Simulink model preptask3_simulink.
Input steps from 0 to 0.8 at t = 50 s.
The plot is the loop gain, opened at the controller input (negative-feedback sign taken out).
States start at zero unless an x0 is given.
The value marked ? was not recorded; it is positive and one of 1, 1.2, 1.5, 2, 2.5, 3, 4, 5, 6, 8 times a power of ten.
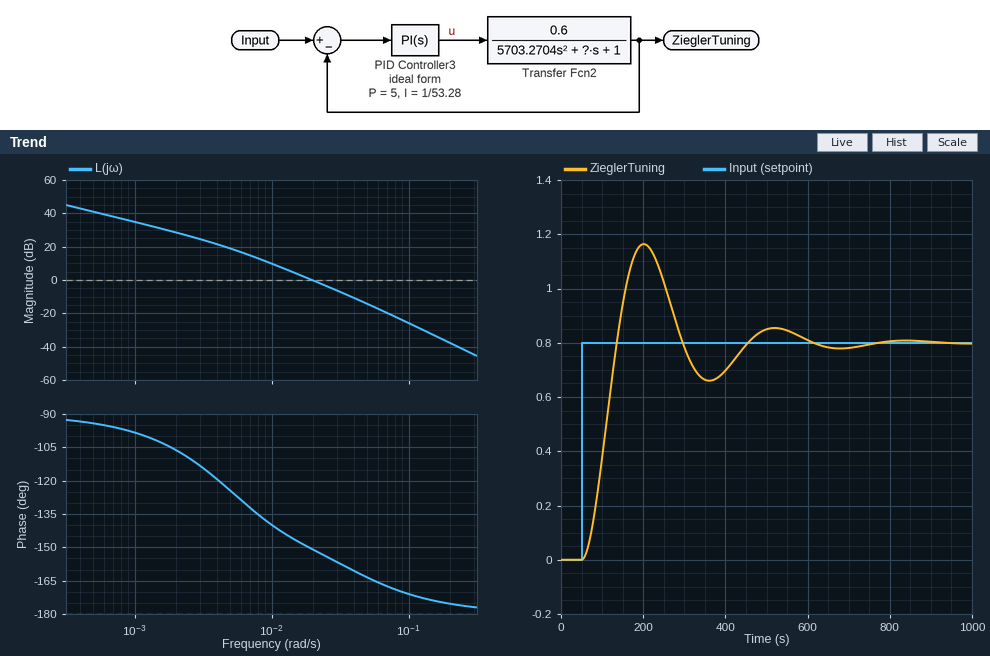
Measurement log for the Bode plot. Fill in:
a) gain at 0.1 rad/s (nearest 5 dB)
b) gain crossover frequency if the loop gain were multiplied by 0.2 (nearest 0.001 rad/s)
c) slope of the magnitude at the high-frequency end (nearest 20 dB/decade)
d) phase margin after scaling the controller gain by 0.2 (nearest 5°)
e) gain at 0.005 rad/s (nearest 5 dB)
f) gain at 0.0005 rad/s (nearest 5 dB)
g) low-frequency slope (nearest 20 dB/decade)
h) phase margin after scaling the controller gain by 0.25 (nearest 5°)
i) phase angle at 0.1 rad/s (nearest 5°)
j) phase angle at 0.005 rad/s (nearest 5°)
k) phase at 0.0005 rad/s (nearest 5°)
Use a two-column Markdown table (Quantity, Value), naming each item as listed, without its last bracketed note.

| Quantity | Value |
|---|---|
| gain at 0.1 rad/s | -25 dB |
| gain crossover frequency if the loop gain were multiplied by 0.2 | 0.007 rad/s |
| slope of the magnitude at the high-frequency end | -40 dB/decade |
| phase margin after scaling the controller gain by 0.2 | 45° |
| gain at 0.005 rad/s | 20 dB |
| gain at 0.0005 rad/s | 40 dB |
| low-frequency slope | -20 dB/decade |
| phase margin after scaling the controller gain by 0.25 | 45° |
| phase angle at 0.1 rad/s | -170° |
| phase angle at 0.005 rad/s | -125° |
| phase at 0.0005 rad/s | -95° |
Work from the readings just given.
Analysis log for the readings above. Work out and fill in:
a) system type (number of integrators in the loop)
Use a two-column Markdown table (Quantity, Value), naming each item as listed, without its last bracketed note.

| Quantity | Value |
|---|---|
| system type | 1 |
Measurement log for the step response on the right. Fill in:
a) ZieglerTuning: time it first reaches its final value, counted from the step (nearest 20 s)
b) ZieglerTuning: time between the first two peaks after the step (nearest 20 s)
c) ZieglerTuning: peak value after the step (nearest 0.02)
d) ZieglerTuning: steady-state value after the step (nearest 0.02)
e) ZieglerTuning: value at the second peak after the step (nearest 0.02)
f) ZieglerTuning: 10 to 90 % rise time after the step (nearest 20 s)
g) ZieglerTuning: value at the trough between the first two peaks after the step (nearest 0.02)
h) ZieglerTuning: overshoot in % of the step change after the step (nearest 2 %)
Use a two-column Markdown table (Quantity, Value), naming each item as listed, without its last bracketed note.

| Quantity | Value |
|---|---|
| ZieglerTuning: time it first reaches its final value, counted from the step | 80 s |
| ZieglerTuning: time between the first two peaks after the step | 320 s |
| ZieglerTuning: peak value after the step | 1.16 |
| ZieglerTuning: steady-state value after the step | 0.80 |
| ZieglerTuning: value at the second peak after the step | 0.86 |
| ZieglerTuning: 10 to 90 % rise time after the step | 60 s |
| ZieglerTuning: value at the trough between the first two peaks after the step | 0.66 |
| ZieglerTuning: overshoot in % of the step change after the step | 46 % |
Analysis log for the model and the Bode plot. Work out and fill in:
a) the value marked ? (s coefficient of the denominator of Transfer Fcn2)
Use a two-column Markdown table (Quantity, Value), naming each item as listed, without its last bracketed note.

| Quantity | Value |
|---|---|
| the value marked ? | 200 |
